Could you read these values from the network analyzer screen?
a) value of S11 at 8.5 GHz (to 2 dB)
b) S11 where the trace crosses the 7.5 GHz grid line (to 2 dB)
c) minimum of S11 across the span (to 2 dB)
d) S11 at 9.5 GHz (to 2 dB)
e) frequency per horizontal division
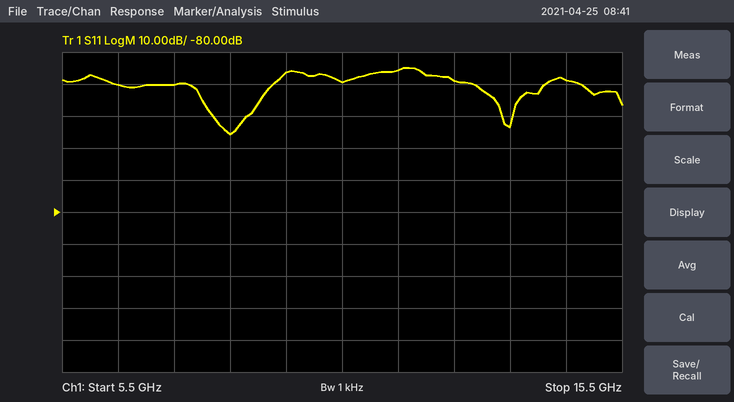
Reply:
-56 dB
-40 dB
-56 dB
-36 dB
1 GHz
